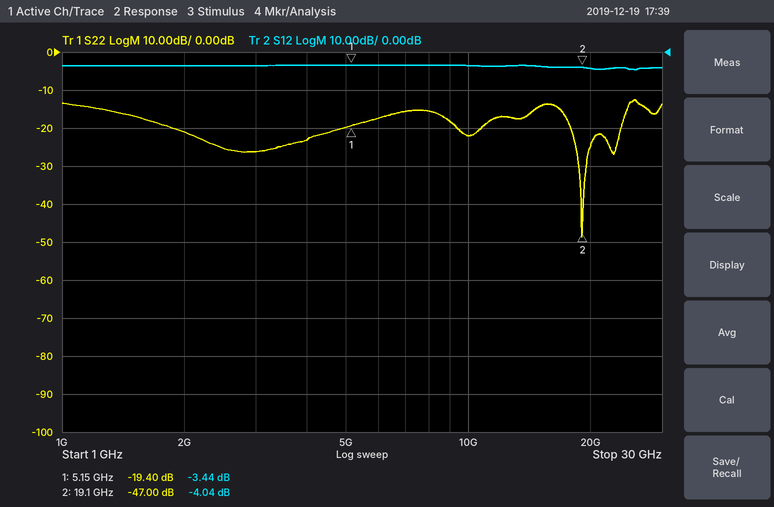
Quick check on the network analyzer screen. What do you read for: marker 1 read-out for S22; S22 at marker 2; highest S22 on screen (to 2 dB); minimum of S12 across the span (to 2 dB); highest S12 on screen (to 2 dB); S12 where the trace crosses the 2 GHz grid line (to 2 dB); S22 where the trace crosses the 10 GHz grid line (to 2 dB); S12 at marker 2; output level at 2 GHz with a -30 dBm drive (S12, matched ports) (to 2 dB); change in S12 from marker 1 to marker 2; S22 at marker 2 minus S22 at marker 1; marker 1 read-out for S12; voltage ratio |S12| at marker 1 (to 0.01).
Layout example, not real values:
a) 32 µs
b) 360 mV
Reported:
a) -19.40 dB
b) -47.00 dB
c) -12 dB
d) -4 dB
e) -4 dB
f) -4 dB
g) -22 dB
h) -4.04 dB
i) -34 dBm
j) -0.60 dB
k) -27.60 dB
l) -3.44 dB
m) 0.67
